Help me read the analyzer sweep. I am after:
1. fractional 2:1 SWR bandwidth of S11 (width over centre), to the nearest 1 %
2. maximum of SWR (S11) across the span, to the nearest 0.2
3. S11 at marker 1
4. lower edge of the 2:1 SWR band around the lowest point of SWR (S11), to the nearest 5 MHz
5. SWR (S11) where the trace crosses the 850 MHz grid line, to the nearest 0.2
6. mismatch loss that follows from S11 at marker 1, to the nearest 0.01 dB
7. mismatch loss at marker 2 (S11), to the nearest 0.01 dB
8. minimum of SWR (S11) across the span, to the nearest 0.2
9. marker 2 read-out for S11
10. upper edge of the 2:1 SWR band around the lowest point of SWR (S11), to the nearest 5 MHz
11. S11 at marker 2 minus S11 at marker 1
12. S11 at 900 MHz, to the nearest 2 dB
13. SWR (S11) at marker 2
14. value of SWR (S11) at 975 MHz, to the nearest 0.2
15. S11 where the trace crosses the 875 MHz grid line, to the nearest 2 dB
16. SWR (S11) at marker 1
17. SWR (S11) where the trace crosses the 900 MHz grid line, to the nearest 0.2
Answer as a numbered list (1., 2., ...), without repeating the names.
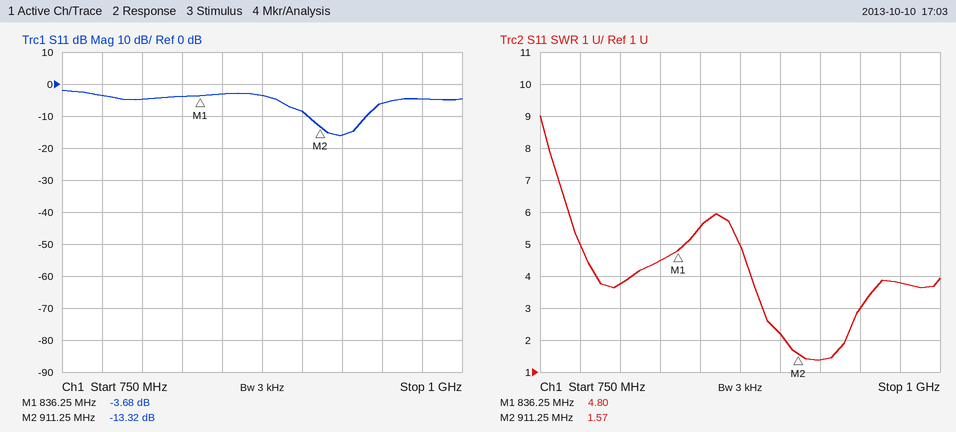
1. 4 %
2. 9.0
3. -3.68 dB
4. 905 MHz
5. 5.6
6. 2.43 dB
7. 0.21 dB
8. 1.4
9. -13.32 dB
10. 940 MHz
11. -9.64 dB
12. -8 dB
13. 1.57
14. 3.8
15. -4 dB
16. 4.80
17. 2.2
